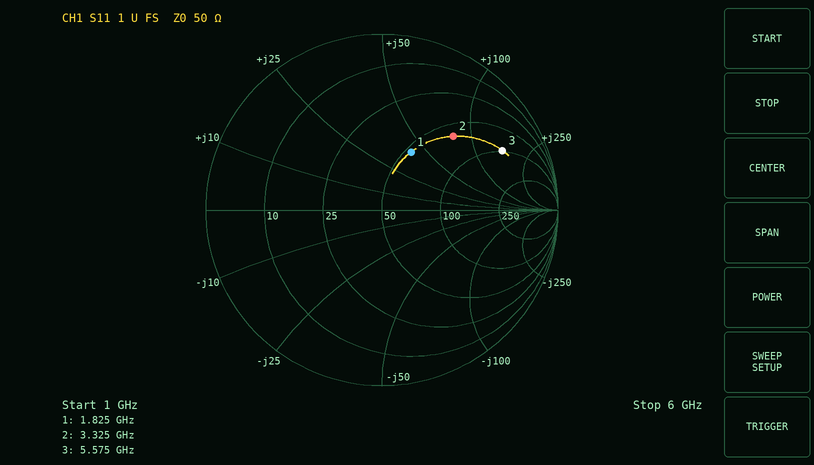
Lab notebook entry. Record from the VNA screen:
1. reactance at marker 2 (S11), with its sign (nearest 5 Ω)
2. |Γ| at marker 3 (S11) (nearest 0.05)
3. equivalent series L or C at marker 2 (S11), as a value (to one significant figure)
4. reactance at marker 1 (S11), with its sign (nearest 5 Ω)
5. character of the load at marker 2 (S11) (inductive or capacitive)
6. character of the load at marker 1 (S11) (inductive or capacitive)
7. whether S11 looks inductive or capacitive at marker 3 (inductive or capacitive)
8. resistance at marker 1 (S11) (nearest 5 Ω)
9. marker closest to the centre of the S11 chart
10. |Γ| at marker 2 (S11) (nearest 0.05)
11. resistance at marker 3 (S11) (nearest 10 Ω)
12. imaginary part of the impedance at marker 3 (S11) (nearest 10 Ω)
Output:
+80 Ω
0.75
4 nH
+40 Ω
inductive
inductive
inductive
55 Ω
marker 1
0.60
100 Ω
+160 Ω
